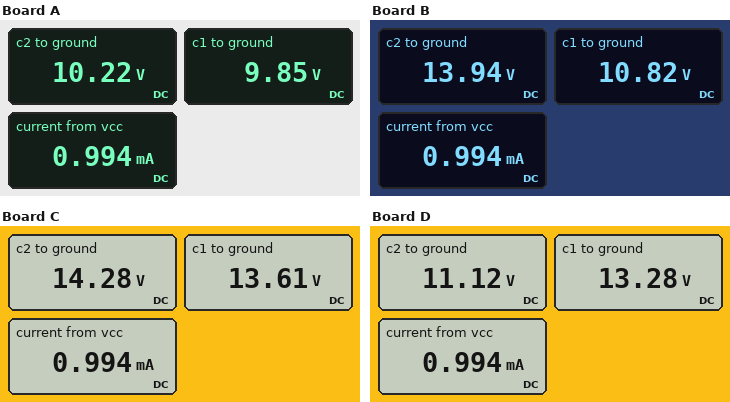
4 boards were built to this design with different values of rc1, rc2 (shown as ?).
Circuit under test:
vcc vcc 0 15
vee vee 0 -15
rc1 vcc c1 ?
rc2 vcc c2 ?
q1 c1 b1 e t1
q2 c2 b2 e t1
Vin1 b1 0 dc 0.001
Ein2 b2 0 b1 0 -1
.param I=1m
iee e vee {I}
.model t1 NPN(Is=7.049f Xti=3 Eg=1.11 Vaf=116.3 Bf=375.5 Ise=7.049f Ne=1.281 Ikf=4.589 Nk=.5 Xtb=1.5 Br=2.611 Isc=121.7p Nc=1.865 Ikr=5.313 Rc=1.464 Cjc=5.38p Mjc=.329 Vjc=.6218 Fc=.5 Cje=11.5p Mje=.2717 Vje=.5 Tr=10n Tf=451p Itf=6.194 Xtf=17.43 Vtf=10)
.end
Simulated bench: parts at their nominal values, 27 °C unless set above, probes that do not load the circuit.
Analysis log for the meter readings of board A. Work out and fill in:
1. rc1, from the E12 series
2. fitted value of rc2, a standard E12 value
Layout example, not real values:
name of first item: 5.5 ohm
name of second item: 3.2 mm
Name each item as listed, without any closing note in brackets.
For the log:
rc1, from the E12 series: 10 kΩ
fitted value of rc2, a standard E12 value: 10 kΩ
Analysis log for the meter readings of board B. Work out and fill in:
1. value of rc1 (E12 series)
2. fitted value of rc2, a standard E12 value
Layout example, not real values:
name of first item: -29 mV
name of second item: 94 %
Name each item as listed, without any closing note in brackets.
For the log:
value of rc1: 8.2 kΩ
fitted value of rc2, a standard E12 value: 2.2 kΩ
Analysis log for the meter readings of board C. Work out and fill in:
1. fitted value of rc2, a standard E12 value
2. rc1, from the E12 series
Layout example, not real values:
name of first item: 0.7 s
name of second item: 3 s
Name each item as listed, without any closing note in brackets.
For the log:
fitted value of rc2, a standard E12 value: 1.5 kΩ
rc1, from the E12 series: 2.7 kΩ
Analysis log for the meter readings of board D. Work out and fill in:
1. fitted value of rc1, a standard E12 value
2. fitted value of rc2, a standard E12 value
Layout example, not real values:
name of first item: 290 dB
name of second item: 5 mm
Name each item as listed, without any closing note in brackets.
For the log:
fitted value of rc1, a standard E12 value: 3.3 kΩ
fitted value of rc2, a standard E12 value: 8.2 kΩ
